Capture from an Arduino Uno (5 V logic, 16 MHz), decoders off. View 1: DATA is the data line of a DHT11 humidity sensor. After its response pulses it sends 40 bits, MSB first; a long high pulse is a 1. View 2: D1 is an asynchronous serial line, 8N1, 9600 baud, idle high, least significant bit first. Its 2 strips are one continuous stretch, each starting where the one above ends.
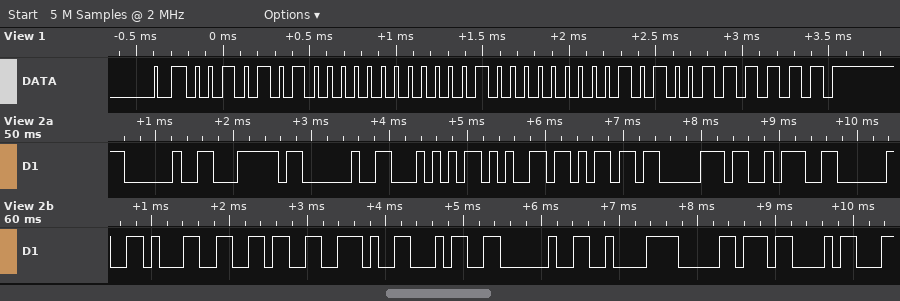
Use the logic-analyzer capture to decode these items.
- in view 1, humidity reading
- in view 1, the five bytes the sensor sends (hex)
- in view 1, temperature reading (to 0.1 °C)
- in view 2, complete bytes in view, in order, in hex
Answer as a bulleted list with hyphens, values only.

- 42 %
- 2A 00 10 05 3F
- 16.5 °C
- 0x20 0x7C 0x20 0x54 0x65 0x6D 0x70 0x3A 0x20 0x31 0x36 0x2E 0x34 0x20 0xC2 0xB0 0x43
